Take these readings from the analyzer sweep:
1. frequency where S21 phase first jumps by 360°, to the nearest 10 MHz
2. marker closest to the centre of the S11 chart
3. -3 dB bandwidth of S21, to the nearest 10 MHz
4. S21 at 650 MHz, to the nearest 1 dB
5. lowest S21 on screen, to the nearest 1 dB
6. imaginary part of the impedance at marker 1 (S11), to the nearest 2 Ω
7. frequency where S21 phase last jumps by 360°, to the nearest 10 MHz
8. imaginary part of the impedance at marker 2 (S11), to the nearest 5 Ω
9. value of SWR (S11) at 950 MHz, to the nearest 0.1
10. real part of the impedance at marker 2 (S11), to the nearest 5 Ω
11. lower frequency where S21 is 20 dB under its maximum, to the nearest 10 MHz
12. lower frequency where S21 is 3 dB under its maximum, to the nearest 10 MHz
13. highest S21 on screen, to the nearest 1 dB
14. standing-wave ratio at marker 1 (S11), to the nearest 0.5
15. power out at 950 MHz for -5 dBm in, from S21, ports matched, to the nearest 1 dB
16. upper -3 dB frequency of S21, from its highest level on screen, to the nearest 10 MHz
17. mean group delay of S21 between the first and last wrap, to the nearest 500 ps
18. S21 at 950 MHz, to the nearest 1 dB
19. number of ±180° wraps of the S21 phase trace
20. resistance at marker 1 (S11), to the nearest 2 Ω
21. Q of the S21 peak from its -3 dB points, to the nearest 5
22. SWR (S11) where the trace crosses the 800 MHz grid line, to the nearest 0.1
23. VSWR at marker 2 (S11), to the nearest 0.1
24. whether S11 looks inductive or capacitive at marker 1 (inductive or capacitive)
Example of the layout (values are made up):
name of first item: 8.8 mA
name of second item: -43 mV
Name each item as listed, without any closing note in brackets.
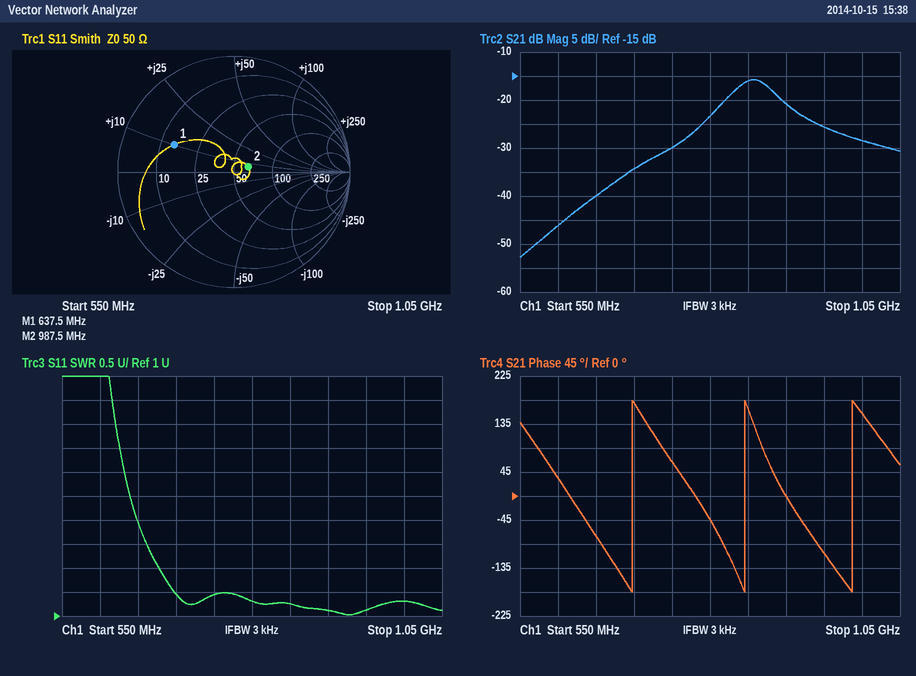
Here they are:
frequency where S21 phase first jumps by 360°, to the nearest 10 MHz: 700 MHz
marker closest to the centre of the S11 chart: marker 2
-3 dB bandwidth of S21, to the nearest 10 MHz: 60 MHz
S21 at 650 MHz, to the nearest 1 dB: -40 dB
lowest S21 on screen, to the nearest 1 dB: -53 dB
imaginary part of the impedance at marker 1 (S11), to the nearest 2 Ω: +10 Ω
frequency where S21 phase last jumps by 360°, to the nearest 10 MHz: 990 MHz
imaginary part of the impedance at marker 2 (S11), to the nearest 5 Ω: +5 Ω
value of SWR (S11) at 950 MHz, to the nearest 0.1: 1.1
real part of the impedance at marker 2 (S11), to the nearest 5 Ω: 65 Ω
lower frequency where S21 is 20 dB under its maximum, to the nearest 10 MHz: 690 MHz
lower frequency where S21 is 3 dB under its maximum, to the nearest 10 MHz: 830 MHz
highest S21 on screen, to the nearest 1 dB: -16 dB
standing-wave ratio at marker 1 (S11), to the nearest 0.5: 3.5
power out at 950 MHz for -5 dBm in, from S21, ports matched, to the nearest 1 dB: -31 dBm
upper -3 dB frequency of S21, from its highest level on screen, to the nearest 10 MHz: 890 MHz
mean group delay of S21 between the first and last wrap, to the nearest 500 ps: 7.0 ns
S21 at 950 MHz, to the nearest 1 dB: -26 dB
number of ±180° wraps of the S21 phase trace: 3
resistance at marker 1 (S11), to the nearest 2 Ω: 14 Ω
Q of the S21 peak from its -3 dB points, to the nearest 5: 15
SWR (S11) where the trace crosses the 800 MHz grid line, to the nearest 0.1: 1.3
VSWR at marker 2 (S11), to the nearest 0.1: 1.3
whether S11 looks inductive or capacitive at marker 1: inductive
